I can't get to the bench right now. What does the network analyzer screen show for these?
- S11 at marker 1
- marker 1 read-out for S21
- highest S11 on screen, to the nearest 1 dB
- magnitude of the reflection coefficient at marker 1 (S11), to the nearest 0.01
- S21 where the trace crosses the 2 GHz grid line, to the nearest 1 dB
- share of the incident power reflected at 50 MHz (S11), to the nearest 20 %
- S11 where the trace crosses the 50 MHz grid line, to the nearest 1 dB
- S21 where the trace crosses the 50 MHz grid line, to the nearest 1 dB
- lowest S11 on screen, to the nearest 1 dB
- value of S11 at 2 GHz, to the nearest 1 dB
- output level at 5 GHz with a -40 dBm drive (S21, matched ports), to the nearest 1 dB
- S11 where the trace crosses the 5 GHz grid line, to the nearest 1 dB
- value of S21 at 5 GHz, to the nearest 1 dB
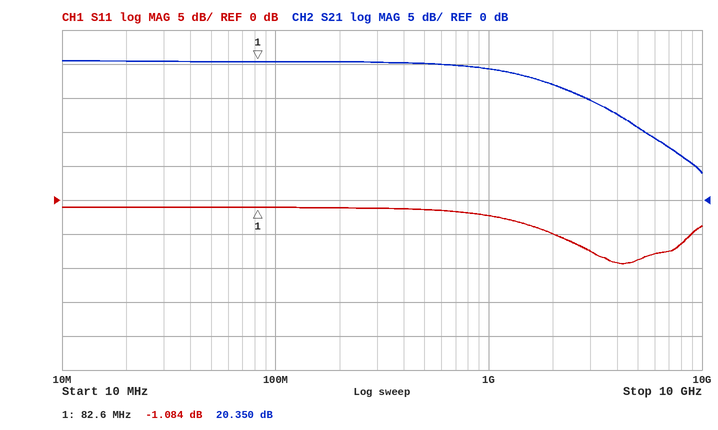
-1.084 dB
20.350 dB
-1 dB
0.88
17 dB
80 %
-1 dB
20 dB
-9 dB
-5 dB
-29 dBm
-9 dB
11 dB
